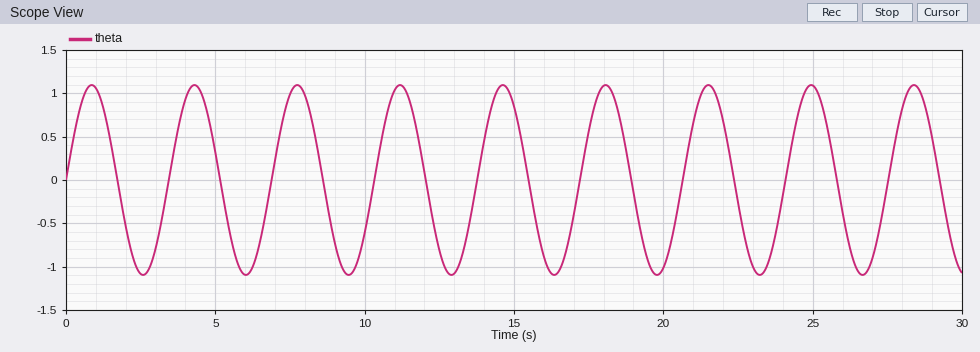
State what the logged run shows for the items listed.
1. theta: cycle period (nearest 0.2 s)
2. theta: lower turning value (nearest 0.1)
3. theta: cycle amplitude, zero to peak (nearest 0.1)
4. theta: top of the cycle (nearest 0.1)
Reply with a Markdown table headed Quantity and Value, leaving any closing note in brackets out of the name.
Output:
| Quantity | Value |
|---|---|
| theta: cycle period | 3.4 s |
| theta: lower turning value | -1.1 |
| theta: cycle amplitude, zero to peak | 1.1 |
| theta: top of the cycle | 1.1 |
